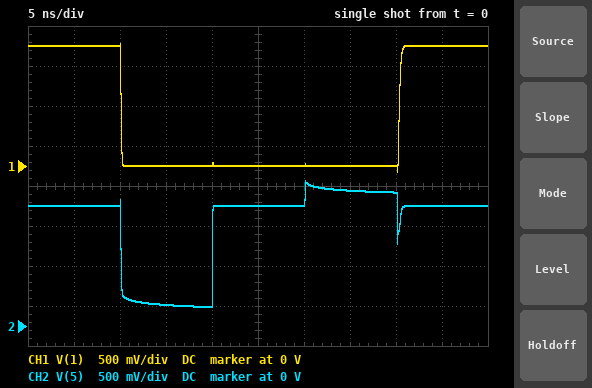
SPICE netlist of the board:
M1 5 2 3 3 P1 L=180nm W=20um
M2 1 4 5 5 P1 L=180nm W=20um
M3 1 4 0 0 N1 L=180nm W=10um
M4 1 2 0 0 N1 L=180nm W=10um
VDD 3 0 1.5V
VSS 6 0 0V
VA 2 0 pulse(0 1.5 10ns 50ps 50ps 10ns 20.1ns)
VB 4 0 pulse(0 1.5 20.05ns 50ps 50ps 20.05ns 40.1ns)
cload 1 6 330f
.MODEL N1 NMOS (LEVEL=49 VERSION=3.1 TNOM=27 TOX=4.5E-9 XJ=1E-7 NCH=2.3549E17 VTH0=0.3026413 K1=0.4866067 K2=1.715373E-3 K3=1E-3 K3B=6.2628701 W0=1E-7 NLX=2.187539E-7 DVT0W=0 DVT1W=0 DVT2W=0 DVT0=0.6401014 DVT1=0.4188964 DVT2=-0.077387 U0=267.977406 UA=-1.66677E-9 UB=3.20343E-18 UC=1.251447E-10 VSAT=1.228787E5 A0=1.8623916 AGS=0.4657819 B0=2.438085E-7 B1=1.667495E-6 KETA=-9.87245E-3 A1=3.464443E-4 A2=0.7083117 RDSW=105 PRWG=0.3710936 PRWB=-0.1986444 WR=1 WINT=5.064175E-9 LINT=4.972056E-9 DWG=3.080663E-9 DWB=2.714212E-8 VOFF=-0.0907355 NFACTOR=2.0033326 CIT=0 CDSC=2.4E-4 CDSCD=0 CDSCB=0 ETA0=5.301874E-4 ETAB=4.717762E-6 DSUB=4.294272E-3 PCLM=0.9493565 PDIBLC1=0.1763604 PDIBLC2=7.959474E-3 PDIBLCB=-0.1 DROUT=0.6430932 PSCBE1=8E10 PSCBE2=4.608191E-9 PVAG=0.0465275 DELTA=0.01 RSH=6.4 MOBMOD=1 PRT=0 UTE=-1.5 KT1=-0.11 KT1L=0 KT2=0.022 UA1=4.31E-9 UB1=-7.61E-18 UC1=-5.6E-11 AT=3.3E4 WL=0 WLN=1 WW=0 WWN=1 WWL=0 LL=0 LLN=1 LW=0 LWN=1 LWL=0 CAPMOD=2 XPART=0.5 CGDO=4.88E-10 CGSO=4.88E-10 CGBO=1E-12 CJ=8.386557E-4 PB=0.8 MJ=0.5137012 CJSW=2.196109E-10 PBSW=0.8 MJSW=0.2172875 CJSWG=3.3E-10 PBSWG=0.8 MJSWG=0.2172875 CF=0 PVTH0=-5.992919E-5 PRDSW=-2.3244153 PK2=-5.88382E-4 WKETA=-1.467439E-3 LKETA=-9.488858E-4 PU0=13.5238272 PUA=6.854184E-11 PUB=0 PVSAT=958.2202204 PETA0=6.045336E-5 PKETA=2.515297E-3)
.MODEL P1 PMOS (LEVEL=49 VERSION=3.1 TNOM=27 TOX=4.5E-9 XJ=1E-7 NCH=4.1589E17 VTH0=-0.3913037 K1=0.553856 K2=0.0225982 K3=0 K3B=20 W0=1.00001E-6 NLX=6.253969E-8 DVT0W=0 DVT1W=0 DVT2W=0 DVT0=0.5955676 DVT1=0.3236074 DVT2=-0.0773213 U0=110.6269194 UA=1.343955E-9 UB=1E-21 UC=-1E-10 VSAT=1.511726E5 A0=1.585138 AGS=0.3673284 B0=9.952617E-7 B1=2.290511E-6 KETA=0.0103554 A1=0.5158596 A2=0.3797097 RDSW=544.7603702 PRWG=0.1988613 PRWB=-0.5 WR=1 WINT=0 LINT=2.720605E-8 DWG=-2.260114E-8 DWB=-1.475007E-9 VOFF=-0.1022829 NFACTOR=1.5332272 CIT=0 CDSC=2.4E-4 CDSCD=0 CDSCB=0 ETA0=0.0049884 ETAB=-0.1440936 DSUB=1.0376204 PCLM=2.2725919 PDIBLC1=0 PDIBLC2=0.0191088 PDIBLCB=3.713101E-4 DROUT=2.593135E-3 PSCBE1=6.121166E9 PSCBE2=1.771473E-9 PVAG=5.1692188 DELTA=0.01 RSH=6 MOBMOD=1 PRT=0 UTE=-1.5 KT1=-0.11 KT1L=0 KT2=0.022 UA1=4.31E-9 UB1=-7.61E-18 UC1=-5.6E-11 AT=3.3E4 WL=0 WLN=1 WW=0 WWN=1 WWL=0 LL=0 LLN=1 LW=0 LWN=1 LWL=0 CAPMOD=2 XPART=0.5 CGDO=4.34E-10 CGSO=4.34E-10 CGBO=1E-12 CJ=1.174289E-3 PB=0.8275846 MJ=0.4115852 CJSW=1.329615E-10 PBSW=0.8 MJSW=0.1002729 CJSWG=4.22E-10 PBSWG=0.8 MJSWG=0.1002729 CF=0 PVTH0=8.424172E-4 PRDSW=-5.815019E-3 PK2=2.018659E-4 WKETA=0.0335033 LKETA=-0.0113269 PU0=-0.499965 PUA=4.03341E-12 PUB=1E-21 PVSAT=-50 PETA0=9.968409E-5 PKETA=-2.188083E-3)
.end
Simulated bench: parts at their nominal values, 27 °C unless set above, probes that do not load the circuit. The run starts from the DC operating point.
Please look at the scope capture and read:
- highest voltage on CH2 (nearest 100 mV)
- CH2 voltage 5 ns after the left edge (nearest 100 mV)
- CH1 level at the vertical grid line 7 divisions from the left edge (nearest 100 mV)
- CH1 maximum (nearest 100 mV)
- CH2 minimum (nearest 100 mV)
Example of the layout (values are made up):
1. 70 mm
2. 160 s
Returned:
1. 1.8 V
2. 1.5 V
3. 0 V
4. 1.5 V
5. 200 mV
